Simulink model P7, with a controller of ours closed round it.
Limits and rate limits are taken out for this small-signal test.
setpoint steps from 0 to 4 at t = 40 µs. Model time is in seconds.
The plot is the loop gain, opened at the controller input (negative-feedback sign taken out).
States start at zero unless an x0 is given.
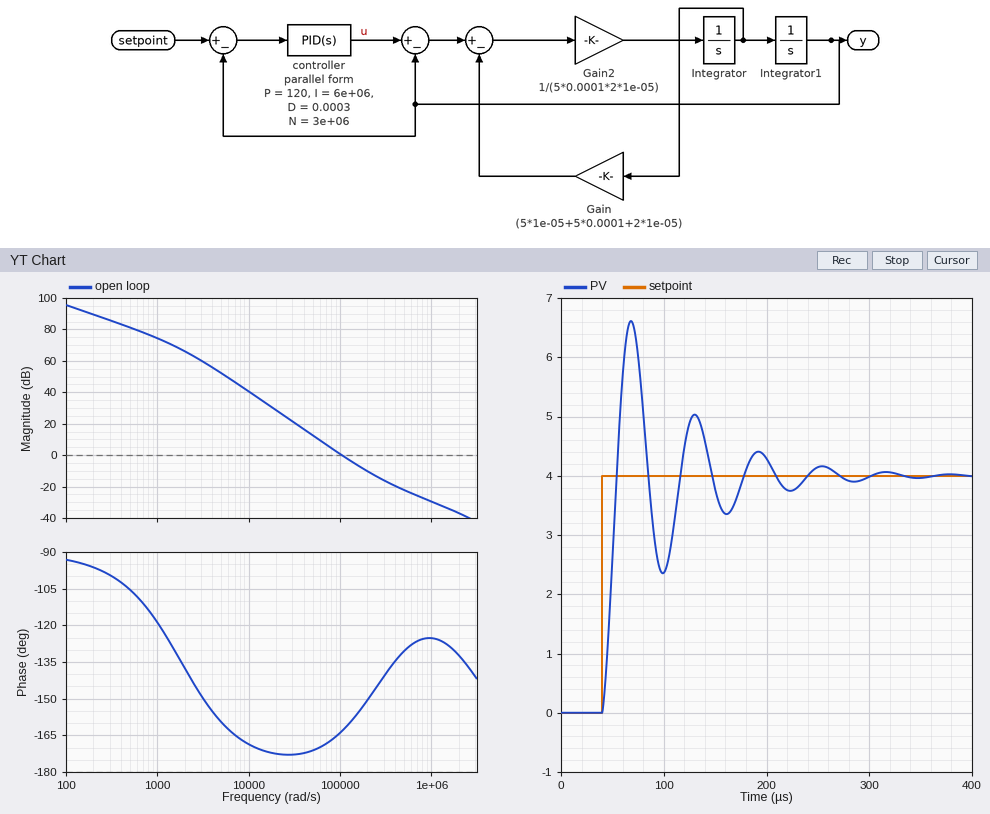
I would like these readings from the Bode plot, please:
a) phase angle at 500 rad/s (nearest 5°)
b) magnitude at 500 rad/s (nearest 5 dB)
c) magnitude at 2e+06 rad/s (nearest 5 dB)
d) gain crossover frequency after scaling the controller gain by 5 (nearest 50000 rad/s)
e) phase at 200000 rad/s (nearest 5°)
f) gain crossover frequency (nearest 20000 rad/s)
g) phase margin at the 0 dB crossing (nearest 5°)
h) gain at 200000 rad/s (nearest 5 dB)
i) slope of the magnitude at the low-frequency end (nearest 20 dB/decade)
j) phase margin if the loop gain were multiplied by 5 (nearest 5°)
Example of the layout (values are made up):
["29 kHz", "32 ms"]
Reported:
["-105°", "80 dB", "-35 dB", "250000 rad/s", "-150°", "100000 rad/s", "15°", "-10 dB", "-20 dB/decade", "35°"]
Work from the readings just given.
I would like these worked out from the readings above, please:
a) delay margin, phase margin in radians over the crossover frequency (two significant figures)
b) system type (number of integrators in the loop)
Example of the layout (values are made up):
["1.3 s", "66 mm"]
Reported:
["0.0000026 s", "1"]
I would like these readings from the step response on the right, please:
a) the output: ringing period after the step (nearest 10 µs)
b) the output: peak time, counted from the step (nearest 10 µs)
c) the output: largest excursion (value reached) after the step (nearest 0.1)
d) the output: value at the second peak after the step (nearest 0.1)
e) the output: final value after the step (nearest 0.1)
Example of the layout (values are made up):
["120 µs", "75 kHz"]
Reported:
["60 µs", "30 µs", "6.6", "5.0", "4.0"]
